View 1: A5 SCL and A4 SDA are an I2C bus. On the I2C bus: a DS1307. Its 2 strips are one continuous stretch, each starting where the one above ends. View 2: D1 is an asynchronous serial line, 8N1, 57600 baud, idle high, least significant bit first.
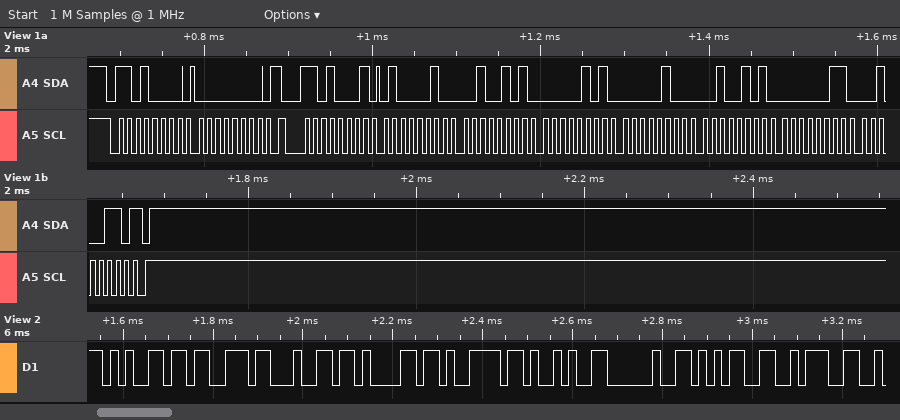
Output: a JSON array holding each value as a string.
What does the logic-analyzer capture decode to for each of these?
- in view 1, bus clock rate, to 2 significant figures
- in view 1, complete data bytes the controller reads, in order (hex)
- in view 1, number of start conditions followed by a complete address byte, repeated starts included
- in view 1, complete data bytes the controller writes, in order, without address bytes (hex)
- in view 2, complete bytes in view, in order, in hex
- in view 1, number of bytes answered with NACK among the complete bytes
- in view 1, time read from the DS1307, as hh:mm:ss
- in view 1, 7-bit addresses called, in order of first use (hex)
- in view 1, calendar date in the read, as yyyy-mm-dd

["100 kHz", "42 25 05 04 25 03 26", "2", "00", "65 73 64 61 79 29 20 35 3A", "1", "05:25:42", "0x68", "2026-03-25"]
